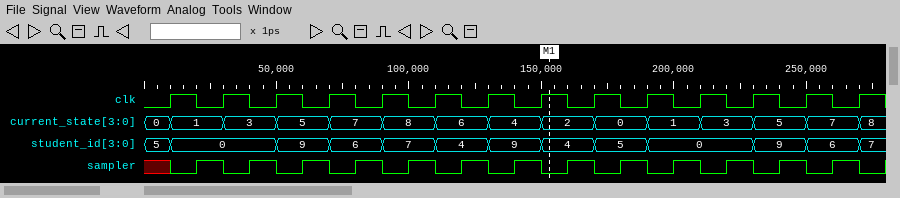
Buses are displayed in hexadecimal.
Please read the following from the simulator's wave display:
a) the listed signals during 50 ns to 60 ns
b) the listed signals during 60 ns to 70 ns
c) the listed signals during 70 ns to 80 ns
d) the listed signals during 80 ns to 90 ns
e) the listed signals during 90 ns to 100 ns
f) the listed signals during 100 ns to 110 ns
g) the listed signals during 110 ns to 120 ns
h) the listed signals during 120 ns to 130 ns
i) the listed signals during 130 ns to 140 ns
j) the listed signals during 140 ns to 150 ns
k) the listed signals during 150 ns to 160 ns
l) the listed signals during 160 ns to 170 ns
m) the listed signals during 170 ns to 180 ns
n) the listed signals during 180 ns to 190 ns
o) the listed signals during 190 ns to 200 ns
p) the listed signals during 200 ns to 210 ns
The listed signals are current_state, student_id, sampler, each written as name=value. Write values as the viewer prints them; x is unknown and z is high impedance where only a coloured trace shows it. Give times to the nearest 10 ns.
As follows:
current_state=5, student_id=9, sampler=0
current_state=5, student_id=9, sampler=1
current_state=7, student_id=6, sampler=0
current_state=7, student_id=6, sampler=1
current_state=8, student_id=7, sampler=0
current_state=8, student_id=7, sampler=1
current_state=6, student_id=4, sampler=0
current_state=6, student_id=4, sampler=1
current_state=4, student_id=9, sampler=0
current_state=4, student_id=9, sampler=1
current_state=2, student_id=4, sampler=0
current_state=2, student_id=4, sampler=1
current_state=0, student_id=5, sampler=0
current_state=0, student_id=5, sampler=1
current_state=1, student_id=0, sampler=0
current_state=1, student_id=0, sampler=1
